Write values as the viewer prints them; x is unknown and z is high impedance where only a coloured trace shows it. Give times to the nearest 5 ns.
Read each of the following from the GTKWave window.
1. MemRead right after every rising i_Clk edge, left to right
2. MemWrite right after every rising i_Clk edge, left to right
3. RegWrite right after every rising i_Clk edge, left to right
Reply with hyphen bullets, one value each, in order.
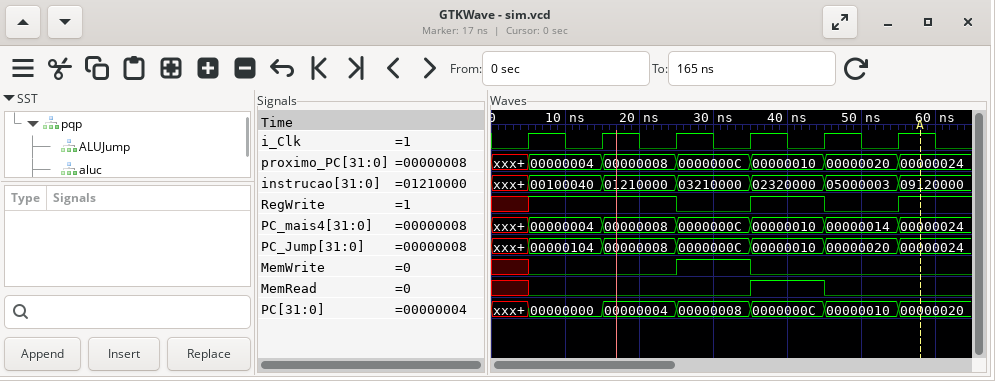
- 0 0 0 1 0 0
- 0 0 1 0 0 0
- 1 1 0 1 0 1
